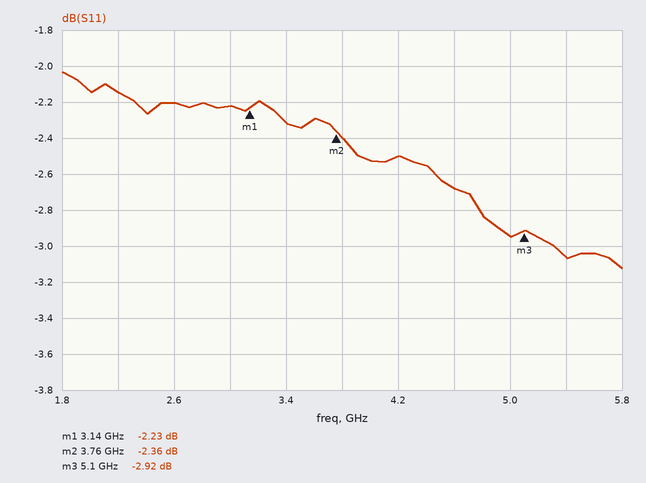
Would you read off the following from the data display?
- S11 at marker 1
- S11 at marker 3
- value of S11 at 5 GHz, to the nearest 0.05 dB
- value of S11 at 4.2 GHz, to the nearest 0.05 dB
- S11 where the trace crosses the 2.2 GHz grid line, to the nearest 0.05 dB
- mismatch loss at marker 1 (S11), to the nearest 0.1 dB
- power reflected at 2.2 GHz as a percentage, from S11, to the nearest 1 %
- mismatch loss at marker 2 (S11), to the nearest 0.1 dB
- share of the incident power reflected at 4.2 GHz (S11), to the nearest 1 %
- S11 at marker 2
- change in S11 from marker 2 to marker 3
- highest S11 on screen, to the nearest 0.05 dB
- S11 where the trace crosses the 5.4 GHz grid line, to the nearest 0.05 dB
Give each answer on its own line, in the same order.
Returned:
-2.23 dB
-2.92 dB
-2.95 dB
-2.50 dB
-2.15 dB
4.0 dB
61 %
3.8 dB
56 %
-2.36 dB
-0.56 dB
-2.05 dB
-3.05 dB
